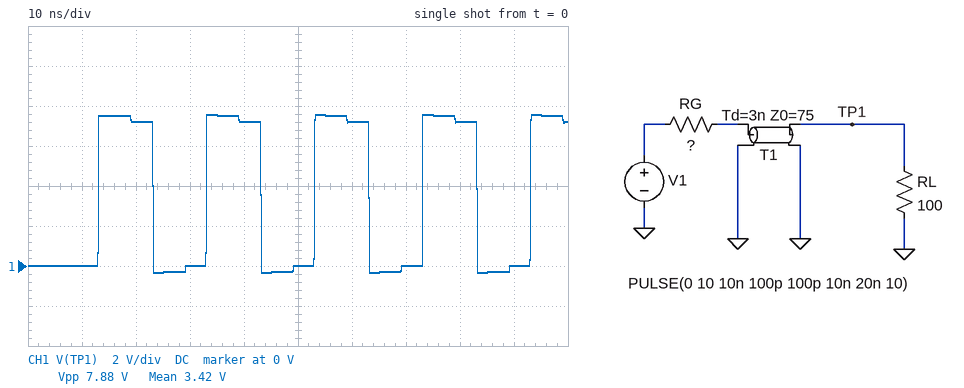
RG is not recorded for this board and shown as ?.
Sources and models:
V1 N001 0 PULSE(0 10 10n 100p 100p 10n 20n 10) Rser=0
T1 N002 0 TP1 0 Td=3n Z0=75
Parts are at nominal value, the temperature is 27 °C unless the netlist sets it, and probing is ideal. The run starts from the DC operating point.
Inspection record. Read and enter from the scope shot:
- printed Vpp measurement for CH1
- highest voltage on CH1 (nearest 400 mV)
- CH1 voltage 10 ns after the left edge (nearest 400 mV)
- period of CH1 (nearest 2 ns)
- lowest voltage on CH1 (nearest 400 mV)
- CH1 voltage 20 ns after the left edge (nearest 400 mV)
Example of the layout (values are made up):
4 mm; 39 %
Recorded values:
7.88 V; 7.6 V; 0 V; 20 ns; -400 mV; 7.2 V
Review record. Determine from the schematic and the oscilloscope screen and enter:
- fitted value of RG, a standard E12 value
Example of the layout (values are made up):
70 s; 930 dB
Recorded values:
39 Ω
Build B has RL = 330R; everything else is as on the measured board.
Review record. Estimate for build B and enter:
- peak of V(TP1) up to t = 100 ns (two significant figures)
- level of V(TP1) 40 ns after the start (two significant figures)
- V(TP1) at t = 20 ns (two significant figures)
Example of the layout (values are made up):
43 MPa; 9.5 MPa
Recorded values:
11 V; 8.5 V; 8.6 V
